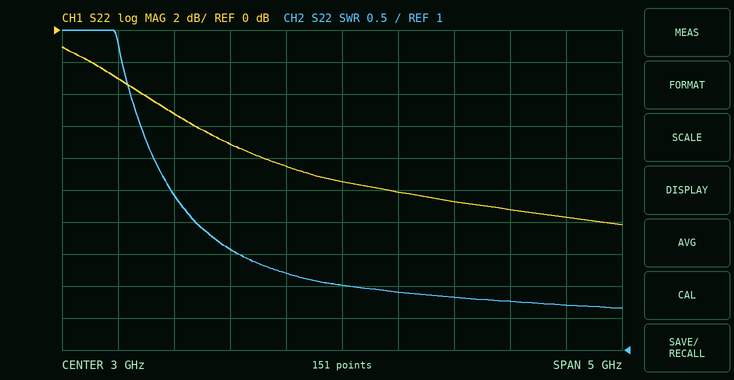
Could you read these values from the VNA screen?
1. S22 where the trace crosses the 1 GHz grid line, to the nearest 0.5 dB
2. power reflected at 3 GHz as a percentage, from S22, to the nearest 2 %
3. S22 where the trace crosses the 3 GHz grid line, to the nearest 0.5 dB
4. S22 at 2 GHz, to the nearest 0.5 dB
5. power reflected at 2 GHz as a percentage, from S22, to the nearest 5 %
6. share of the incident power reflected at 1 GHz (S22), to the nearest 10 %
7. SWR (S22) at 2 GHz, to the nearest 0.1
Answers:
-3.0 dB
12 %
-9.5 dB
-7.0 dB
20 %
50 %
2.6
